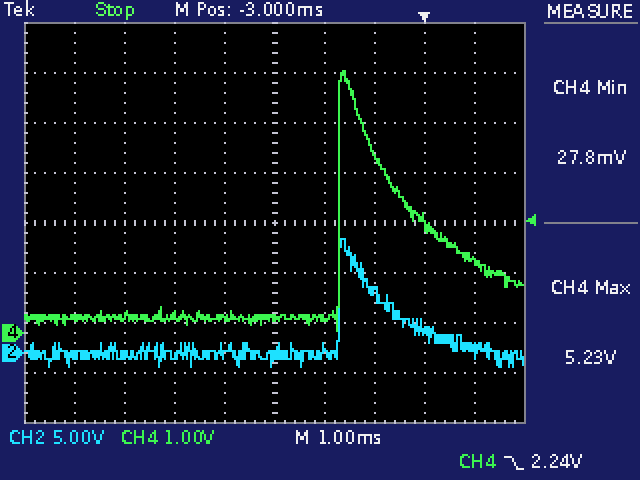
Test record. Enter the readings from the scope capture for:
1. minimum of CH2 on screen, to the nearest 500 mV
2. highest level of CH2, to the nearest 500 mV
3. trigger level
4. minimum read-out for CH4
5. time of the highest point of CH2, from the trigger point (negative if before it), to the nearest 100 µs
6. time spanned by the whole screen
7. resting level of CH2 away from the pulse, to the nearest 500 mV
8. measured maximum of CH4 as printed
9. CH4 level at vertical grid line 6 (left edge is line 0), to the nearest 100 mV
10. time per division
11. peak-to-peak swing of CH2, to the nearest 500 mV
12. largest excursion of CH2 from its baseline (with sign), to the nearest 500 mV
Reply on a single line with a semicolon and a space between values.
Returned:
-1.5 V; 11.5 V; 2.24 V; 27.8 mV; -1.6 ms; 10 ms; 0.0 V; 5.23 V; 300 mV; 1 ms; 13.0 V; +11.5 V
